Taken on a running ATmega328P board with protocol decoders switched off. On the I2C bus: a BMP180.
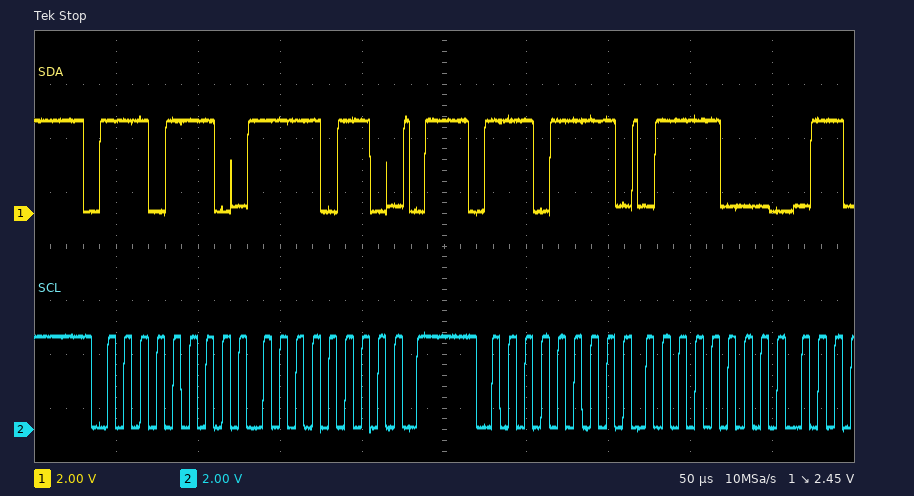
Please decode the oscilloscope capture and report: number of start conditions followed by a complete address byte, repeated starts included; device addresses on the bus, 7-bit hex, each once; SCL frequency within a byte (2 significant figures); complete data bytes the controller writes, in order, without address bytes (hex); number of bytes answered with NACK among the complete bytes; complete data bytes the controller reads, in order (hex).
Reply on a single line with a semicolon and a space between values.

2; 0x77; 100 kHz; F6; 0; 78
